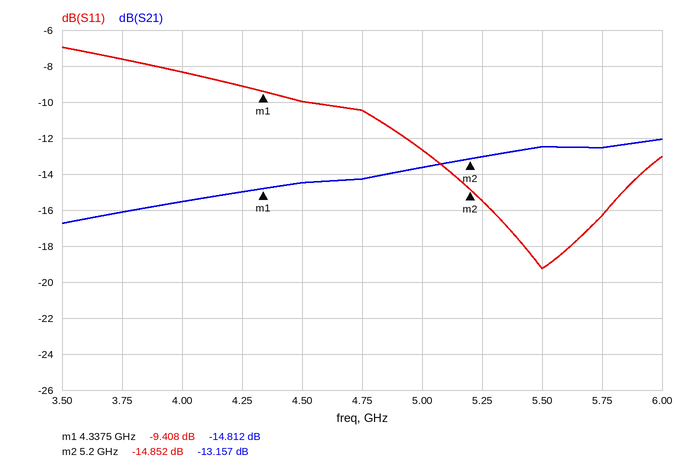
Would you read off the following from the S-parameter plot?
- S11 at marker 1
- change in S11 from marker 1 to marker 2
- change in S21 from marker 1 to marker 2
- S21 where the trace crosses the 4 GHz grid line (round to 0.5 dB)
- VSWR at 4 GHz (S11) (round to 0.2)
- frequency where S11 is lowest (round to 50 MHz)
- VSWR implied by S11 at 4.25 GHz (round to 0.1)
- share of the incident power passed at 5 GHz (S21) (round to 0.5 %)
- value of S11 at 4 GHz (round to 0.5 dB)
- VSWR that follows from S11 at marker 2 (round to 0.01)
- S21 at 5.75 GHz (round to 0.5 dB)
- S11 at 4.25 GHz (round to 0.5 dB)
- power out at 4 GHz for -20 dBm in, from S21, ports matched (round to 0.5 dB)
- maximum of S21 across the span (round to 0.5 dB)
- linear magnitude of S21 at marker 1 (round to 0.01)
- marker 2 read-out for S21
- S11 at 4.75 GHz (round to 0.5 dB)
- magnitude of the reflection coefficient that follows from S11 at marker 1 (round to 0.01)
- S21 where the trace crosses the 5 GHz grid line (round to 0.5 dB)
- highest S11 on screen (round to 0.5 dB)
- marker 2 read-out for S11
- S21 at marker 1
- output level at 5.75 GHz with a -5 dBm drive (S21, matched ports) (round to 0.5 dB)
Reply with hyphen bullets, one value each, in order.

- -9.408 dB
- -5.444 dB
- 1.655 dB
- -15.5 dB
- 2.2
- 5.50 GHz
- 2.1
- 4.5 %
- -8.5 dB
- 1.44
- -12.5 dB
- -9.0 dB
- -35.5 dBm
- -12.0 dB
- 0.18
- -13.157 dB
- -10.5 dB
- 0.34
- -13.5 dB
- -7.0 dB
- -14.852 dB
- -14.812 dB
- -17.5 dBm
